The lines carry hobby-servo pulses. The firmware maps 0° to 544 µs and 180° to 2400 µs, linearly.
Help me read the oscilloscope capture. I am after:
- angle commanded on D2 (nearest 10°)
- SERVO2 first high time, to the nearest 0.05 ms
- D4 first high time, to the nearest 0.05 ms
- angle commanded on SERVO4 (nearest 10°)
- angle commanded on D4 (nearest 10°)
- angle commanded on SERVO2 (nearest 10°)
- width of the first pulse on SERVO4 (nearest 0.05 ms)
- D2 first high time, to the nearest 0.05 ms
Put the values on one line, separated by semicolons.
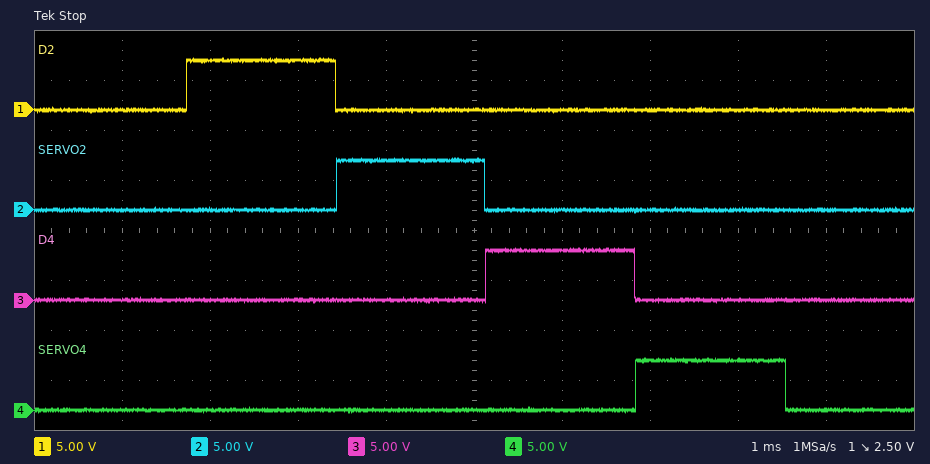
110°; 1.70 ms; 1.70 ms; 110°; 110°; 110°; 1.70 ms; 1.70 ms
